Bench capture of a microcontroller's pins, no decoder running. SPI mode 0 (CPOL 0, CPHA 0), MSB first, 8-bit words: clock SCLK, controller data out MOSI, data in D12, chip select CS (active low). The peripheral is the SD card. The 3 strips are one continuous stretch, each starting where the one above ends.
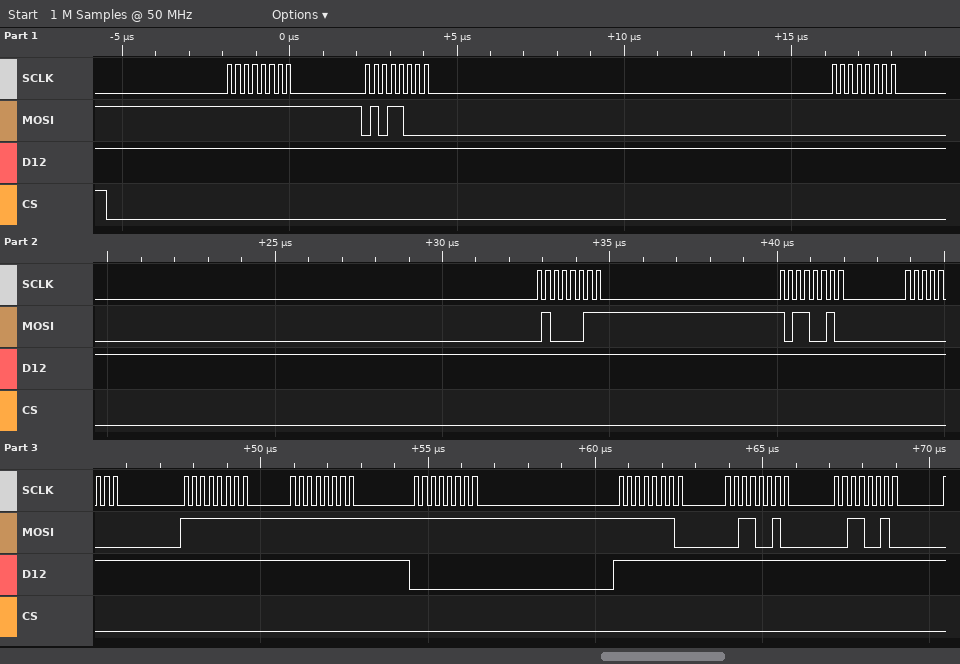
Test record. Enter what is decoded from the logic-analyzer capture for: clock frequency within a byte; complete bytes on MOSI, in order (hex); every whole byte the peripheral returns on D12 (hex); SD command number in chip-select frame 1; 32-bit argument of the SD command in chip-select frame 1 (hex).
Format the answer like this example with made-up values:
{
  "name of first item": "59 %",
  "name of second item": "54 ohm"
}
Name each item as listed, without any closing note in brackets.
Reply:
{
  "clock frequency within a byte": "4 MHz",
  "complete bytes on MOSI, in order": "0xFF 0x58 0x00 0x43 0xB2 0x00 0xFF 0xFF 0xFF 0xFE 0x32 0x32",
  "every whole byte the peripheral returns on D12": "0xFF 0xFF 0xFF 0xFF 0xFF 0xFF 0xFF 0xFF 0x00 0xFF 0xFF 0xFF",
  "SD command number in chip-select frame 1": "CMD24",
  "32-bit argument of the SD command in chip-select frame 1": "0x0043B200"
}
